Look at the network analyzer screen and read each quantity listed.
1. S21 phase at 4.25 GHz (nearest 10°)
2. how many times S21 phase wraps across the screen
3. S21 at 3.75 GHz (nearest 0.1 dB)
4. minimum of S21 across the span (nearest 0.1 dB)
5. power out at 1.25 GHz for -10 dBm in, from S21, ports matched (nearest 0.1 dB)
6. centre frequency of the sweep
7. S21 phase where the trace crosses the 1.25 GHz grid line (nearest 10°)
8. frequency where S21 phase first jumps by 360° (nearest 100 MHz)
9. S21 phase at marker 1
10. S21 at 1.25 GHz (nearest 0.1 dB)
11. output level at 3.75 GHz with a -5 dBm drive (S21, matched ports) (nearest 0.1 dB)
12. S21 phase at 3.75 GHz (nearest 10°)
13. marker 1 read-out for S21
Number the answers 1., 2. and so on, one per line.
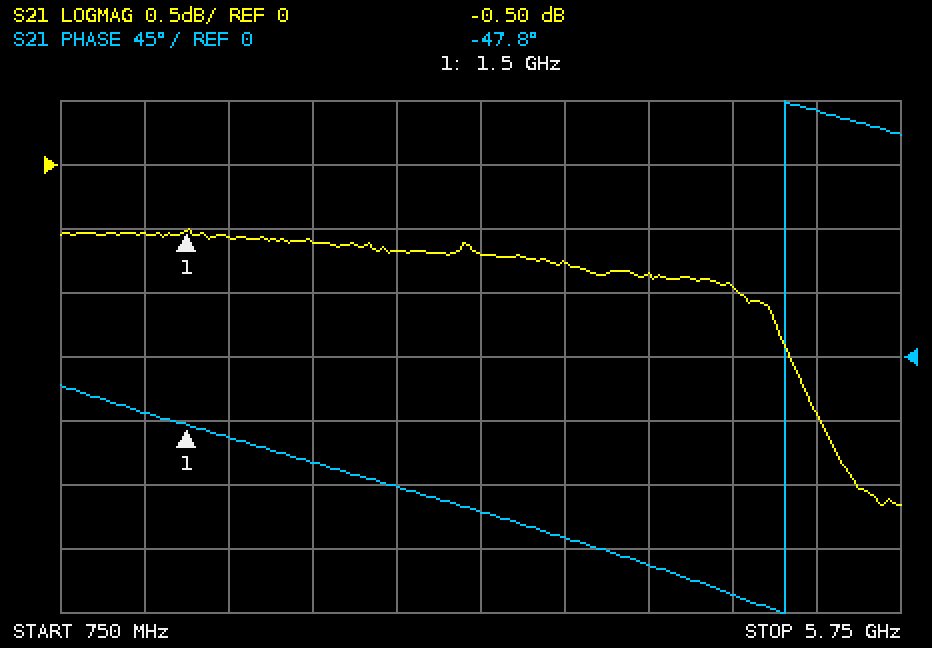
1. -150°
2. 1
3. -0.8 dB
4. -2.7 dB
5. -10.5 dBm
6. 3.25 GHz
7. -40°
8. 5.1 GHz
9. -47.8°
10. -0.5 dB
11. -5.8 dBm
12. -130°
13. -0.50 dB
